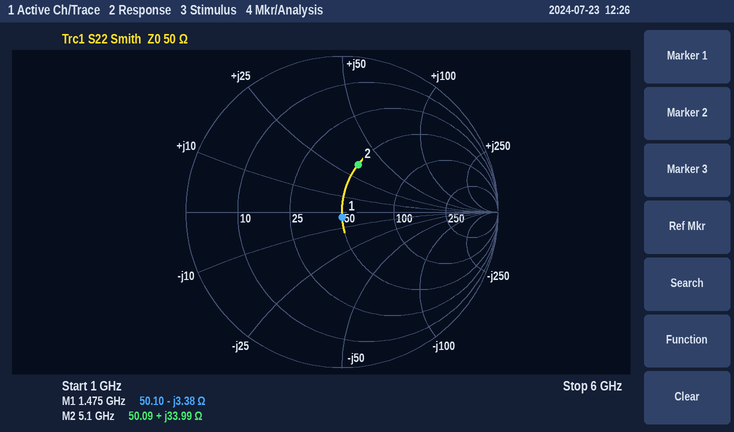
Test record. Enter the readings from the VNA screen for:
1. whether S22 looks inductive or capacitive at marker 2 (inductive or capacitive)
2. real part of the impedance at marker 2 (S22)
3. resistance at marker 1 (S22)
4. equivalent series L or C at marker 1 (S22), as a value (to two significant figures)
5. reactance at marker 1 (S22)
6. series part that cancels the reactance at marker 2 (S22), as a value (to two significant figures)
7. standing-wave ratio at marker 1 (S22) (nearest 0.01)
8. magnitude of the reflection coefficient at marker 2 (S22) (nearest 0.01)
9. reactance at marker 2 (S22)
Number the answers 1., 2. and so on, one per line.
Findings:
1. inductive
2. 50.09 Ω
3. 50.10 Ω
4. 32 pF
5. -3.38 Ω
6. 920 fF
7. 1.07
8. 0.32
9. +33.99 Ω
